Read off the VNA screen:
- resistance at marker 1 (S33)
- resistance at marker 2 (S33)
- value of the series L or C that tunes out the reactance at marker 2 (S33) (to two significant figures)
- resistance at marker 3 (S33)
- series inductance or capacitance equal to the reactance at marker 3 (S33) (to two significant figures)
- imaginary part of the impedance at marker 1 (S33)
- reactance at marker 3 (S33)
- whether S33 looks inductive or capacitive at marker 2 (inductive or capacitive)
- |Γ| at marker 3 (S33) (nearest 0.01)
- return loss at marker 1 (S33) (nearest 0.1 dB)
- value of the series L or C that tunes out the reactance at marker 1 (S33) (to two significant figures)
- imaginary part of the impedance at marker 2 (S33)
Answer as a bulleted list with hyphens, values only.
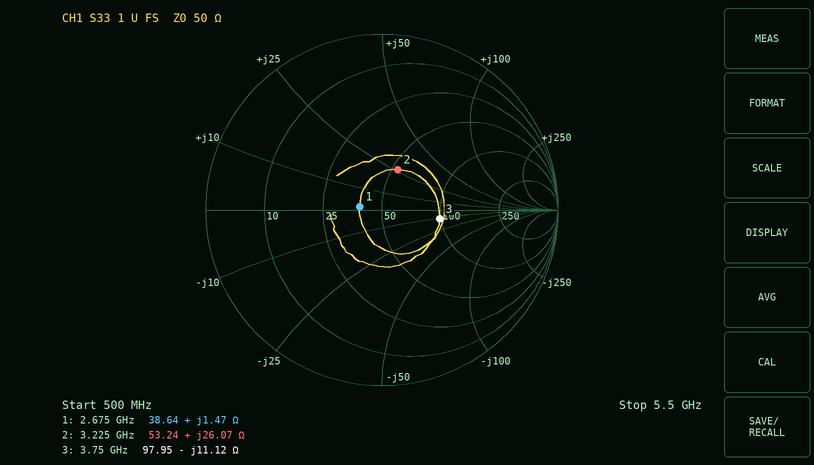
- 38.64 Ω
- 53.24 Ω
- 1.9 pF
- 97.95 Ω
- 3.8 pF
- +1.47 Ω
- -11.12 Ω
- inductive
- 0.33
- 17.8 dB
- 40 pF
- +26.07 Ω
